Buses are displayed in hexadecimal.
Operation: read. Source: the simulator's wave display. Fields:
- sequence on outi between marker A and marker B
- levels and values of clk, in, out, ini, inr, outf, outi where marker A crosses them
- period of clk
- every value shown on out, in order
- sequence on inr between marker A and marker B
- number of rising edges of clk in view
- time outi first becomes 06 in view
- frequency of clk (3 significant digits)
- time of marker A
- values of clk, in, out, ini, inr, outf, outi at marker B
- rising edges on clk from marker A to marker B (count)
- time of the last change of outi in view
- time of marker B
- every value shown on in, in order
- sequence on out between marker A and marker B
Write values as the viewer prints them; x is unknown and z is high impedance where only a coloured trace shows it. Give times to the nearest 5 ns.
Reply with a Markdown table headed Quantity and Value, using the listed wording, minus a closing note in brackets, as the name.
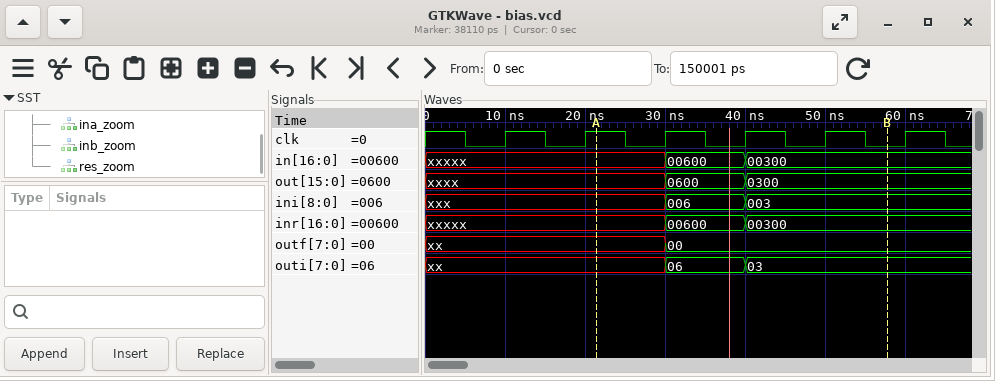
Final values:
| Quantity | Value |
|---|---|
| sequence on outi between marker A and marker B | xx, 06, 03 |
| levels and values of clk, in, out, ini, inr, outf, outi where marker A crosses them | clk=1, in=xxxxx, out=xxxx, ini=xxx, inr=xxxxx, outf=xx, outi=xx |
| period of clk | 10 ns |
| every value shown on out, in order | xxxx, 0600, 0300 |
| sequence on inr between marker A and marker B | xxxxx, 00600, 00300 |
| number of rising edges of clk in view | 6 |
| time outi first becomes 06 in view | 30 ns |
| frequency of clk | 100 MHz |
| time of marker A | 20 ns |
| values of clk, in, out, ini, inr, outf, outi at marker B | clk=0, in=00300, out=0300, ini=003, inr=00300, outf=00, outi=03 |
| rising edges on clk from marker A to marker B | 3 |
| time of the last change of outi in view | 40 ns |
| time of marker B | 60 ns |
| every value shown on in, in order | xxxxx, 00600, 00300 |
| sequence on out between marker A and marker B | xxxx, 0600, 0300 |
